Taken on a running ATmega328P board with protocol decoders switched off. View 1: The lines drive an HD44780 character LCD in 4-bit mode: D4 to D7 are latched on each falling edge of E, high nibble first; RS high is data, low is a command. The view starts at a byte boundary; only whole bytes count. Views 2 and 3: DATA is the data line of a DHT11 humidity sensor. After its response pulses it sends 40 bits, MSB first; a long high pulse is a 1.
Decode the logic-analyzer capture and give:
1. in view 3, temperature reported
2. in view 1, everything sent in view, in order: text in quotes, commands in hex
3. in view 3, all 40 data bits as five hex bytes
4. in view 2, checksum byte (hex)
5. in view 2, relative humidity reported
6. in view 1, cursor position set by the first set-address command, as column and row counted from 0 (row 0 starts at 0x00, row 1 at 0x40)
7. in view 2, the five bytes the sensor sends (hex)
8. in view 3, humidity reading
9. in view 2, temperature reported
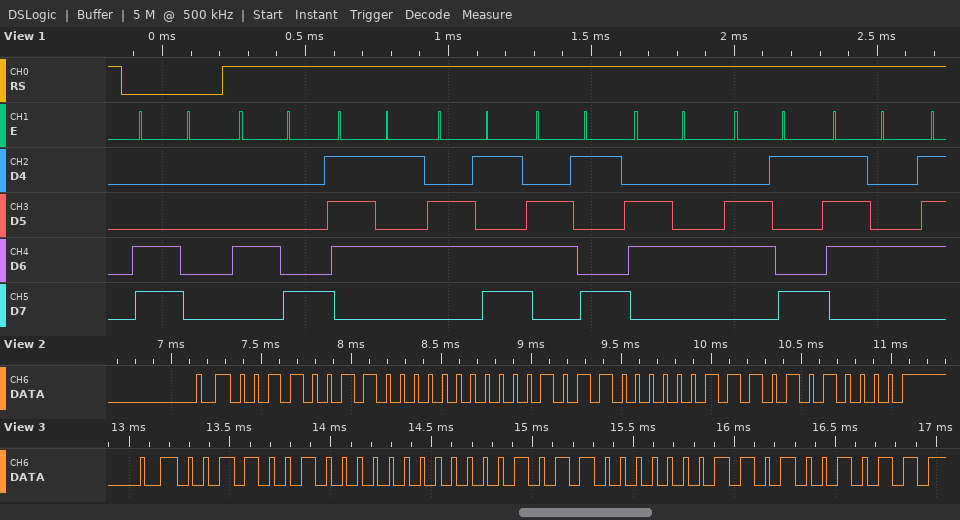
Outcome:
22.3 °C
0xC0 "Humidit"
32 00 16 03 4B
0x50
51 %
column 0, row 1
33 00 16 07 50
50 %
22.7 °C
